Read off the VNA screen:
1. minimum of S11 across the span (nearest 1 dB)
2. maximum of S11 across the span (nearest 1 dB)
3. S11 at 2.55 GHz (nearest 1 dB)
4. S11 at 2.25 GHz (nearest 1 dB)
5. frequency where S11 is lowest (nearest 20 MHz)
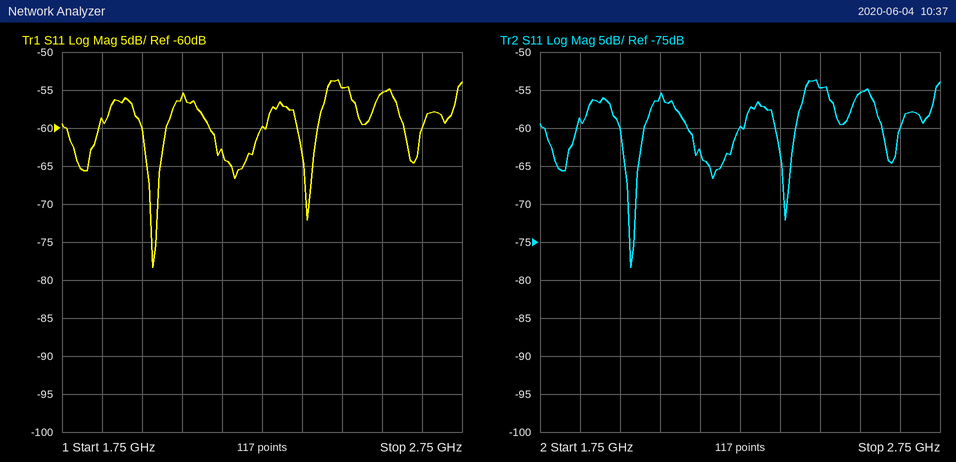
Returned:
-78 dB
-54 dB
-55 dB
-60 dB
1.98 GHz
